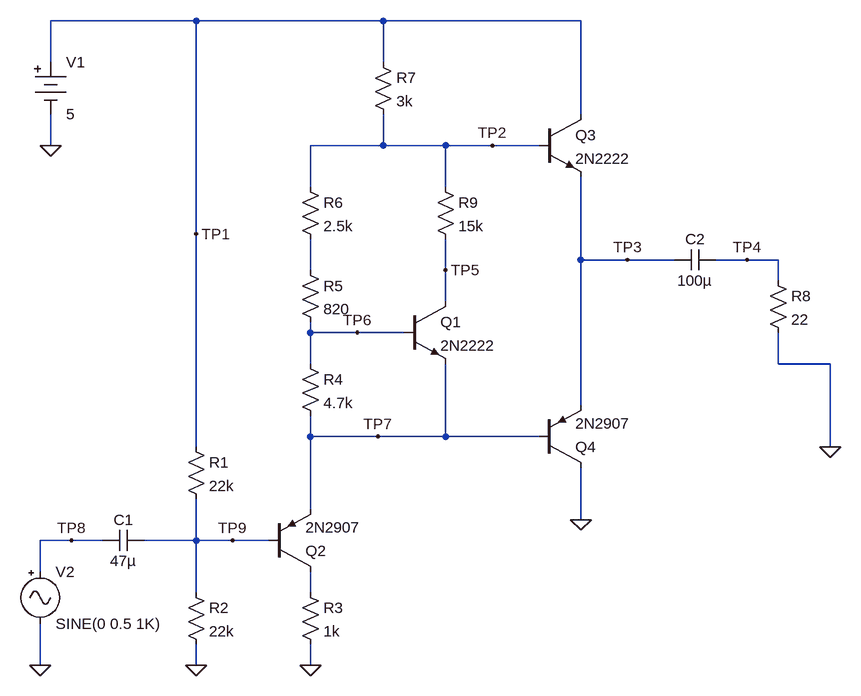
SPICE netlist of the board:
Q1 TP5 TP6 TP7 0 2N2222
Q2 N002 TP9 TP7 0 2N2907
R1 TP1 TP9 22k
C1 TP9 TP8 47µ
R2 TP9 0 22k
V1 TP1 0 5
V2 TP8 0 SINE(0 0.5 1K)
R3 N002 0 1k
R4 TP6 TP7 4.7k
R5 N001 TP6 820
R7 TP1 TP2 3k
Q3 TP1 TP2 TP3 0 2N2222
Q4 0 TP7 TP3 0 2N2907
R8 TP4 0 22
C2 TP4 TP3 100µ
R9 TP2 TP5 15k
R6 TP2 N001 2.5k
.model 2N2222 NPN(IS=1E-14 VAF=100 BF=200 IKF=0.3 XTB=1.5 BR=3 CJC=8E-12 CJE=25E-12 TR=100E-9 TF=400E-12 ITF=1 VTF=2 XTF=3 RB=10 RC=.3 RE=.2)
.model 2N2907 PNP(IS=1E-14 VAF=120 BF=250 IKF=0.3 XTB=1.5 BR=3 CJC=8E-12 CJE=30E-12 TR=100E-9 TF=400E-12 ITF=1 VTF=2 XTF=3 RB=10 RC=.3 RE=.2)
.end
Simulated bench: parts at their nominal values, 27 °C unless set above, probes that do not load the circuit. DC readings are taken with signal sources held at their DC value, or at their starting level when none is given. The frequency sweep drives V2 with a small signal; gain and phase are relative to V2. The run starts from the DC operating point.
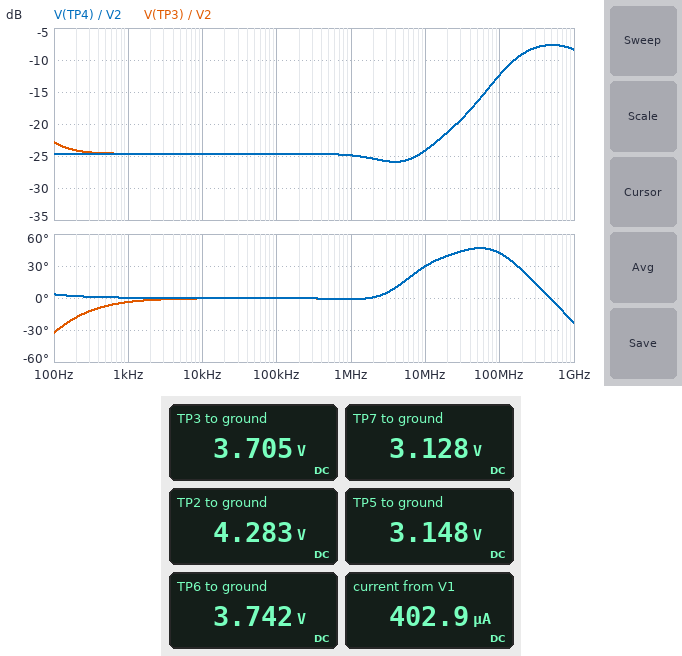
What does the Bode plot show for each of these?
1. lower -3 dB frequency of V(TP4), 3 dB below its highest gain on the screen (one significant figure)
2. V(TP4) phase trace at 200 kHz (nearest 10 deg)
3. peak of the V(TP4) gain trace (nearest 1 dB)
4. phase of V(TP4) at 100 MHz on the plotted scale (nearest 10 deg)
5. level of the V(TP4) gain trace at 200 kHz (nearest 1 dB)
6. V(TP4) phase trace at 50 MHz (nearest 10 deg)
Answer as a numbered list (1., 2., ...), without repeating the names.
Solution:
1. 100 MHz
2. 0 deg
3. -8 dB
4. 40 deg
5. -25 dB
6. 50 deg
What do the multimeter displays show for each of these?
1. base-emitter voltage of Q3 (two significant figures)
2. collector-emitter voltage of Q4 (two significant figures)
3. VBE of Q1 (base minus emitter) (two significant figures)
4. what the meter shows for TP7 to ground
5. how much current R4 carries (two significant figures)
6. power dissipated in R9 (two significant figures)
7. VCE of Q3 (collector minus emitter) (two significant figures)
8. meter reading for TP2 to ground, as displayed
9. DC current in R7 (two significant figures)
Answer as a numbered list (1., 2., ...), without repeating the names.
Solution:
1. 580 mV
2. -3.7 V
3. 610 mV
4. 3.128 V
5. 130 µA
6. 86 µW
7. 1.3 V
8. 4.283 V
9. 240 µA
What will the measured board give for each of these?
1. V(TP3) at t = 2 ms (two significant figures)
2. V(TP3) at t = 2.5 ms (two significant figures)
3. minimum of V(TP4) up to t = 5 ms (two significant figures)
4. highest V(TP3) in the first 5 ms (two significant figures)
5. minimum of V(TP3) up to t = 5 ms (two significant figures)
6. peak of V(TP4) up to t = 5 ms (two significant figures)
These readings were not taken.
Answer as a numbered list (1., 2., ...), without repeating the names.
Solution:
1. 3.7 V
2. 3.7 V
3. -330 mV
4. 3.8 V
5. 3.4 V
6. 170 mV
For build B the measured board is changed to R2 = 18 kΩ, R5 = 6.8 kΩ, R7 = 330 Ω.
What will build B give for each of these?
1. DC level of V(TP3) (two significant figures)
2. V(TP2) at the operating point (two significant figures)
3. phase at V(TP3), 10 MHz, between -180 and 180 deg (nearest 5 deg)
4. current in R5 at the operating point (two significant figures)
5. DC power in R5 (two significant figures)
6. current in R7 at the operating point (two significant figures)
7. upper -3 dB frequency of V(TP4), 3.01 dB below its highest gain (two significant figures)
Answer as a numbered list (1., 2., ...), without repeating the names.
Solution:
1. 3.8 V
2. 4.6 V
3. -5 deg
4. 120 µA
5. 96 µW
6. 1.2 mA
7. 100 MHz
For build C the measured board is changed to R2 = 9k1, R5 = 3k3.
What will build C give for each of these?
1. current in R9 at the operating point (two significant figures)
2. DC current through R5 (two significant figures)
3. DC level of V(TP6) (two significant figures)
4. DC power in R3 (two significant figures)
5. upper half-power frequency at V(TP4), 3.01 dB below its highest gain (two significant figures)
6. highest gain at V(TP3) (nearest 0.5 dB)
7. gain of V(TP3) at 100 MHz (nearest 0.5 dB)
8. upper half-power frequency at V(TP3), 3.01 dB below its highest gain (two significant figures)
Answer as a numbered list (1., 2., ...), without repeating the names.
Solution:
1. 100 µA
2. 160 µA
3. 2.7 V
4. 170 µW
5. 63 MHz
6. -0.5 dB
7. -4.5 dB
8. 54 MHz
